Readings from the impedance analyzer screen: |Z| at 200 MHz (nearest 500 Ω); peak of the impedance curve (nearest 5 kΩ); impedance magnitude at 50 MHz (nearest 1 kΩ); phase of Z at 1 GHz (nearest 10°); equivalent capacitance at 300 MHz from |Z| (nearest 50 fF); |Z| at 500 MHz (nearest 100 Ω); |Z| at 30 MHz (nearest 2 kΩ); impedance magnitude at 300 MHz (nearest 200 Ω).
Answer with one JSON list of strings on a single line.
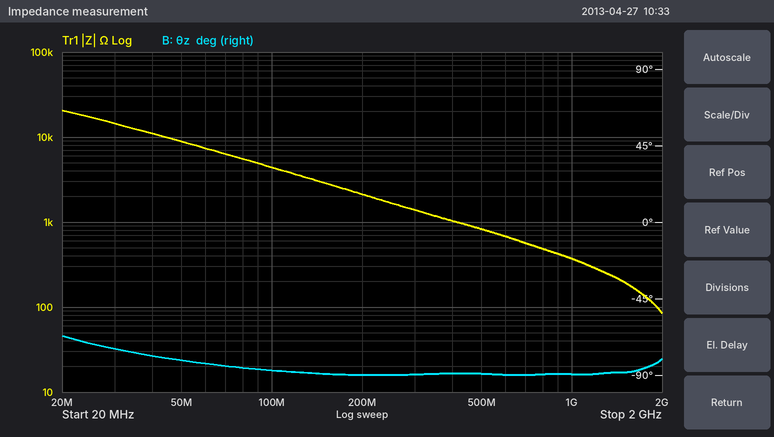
["2.0 kΩ", "20 kΩ", "9 kΩ", "-90°", "400 fF", "800 Ω", "14 kΩ", "1.4 kΩ"]
